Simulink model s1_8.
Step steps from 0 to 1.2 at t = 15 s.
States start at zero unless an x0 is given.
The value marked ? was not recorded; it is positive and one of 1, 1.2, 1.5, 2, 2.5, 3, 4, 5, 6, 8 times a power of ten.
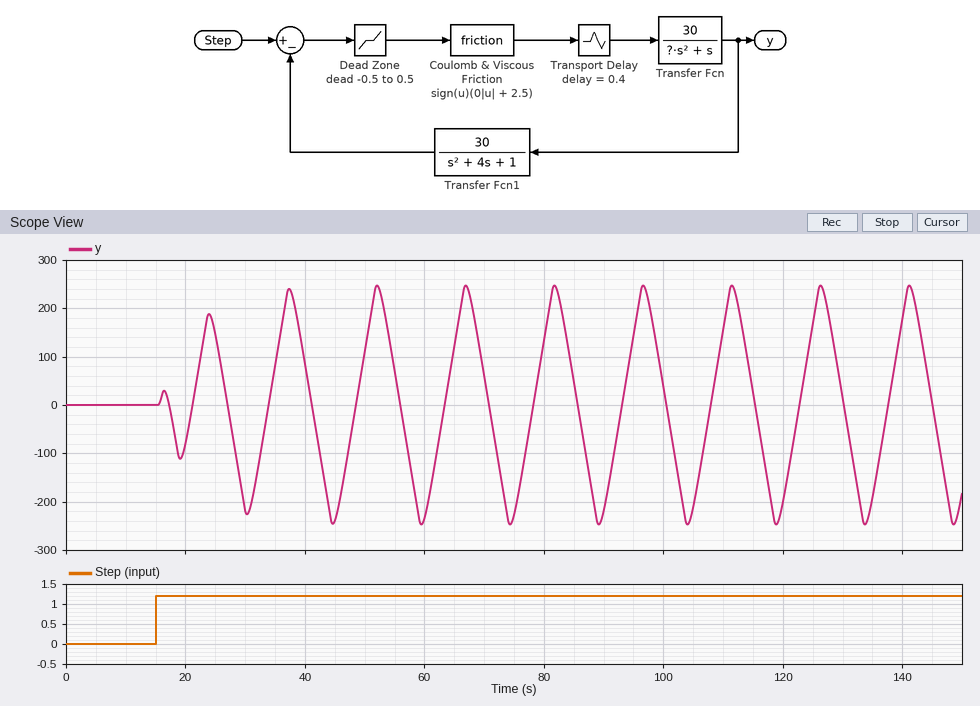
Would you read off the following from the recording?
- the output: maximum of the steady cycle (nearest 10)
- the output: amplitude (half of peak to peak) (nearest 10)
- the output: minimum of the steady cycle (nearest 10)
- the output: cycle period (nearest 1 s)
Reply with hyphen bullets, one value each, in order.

- 250
- 250
- -250
- 15 s
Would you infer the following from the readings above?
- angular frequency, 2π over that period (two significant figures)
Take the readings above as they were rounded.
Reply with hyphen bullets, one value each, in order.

- 0.42 rad/s
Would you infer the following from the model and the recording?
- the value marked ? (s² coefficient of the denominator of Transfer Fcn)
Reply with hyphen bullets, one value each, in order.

- 0.6
